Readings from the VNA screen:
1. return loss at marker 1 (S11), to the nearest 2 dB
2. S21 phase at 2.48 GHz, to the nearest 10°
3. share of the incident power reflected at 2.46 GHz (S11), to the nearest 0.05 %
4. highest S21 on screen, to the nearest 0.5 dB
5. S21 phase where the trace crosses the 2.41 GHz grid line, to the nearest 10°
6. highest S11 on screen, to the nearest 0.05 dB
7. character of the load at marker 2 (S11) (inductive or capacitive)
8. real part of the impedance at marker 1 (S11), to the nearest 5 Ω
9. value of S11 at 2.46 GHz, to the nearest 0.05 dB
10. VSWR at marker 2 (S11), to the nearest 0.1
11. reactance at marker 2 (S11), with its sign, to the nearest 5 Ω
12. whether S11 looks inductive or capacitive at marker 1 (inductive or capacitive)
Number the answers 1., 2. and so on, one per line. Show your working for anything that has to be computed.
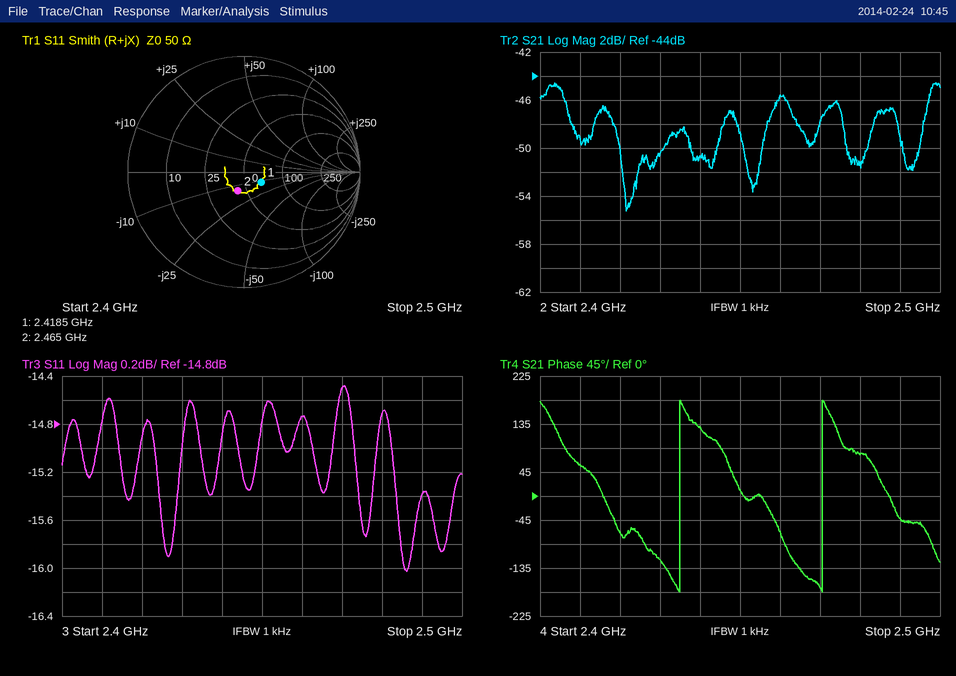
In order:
1. 16 dB
2. 80°
3. 10^(-14.75/10) ≈ 3.35 %
4. -44.5 dB
5. 60°
6. -14.50 dB
7. capacitive
8. 65 Ω
9. -14.75 dB
10. 1.4
11. -15 Ω
12. capacitive
